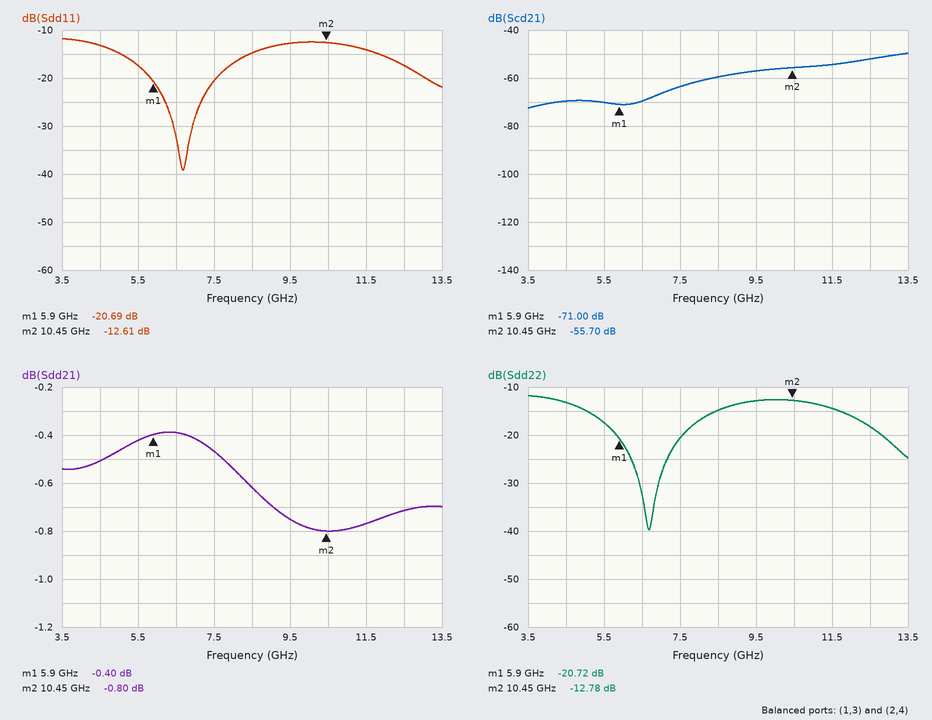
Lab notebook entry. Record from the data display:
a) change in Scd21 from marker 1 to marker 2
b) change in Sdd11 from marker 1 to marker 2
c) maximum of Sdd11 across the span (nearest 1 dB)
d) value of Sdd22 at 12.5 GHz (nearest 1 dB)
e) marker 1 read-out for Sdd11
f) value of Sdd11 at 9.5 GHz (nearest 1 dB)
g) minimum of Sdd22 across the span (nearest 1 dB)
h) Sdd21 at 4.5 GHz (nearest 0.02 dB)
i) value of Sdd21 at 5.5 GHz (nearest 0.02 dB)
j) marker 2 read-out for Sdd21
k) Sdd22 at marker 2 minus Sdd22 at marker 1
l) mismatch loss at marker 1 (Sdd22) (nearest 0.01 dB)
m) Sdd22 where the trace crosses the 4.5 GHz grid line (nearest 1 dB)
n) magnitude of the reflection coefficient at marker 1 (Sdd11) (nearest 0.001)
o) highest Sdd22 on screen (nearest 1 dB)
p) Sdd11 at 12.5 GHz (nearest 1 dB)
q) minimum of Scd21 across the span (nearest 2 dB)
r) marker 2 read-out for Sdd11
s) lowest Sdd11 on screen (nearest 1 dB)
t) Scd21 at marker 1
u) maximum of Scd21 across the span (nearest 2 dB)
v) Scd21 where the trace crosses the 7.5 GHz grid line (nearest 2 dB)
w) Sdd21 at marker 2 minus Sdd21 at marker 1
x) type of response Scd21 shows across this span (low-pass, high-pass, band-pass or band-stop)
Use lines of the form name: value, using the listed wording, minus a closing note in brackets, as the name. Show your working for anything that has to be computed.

change in Scd21 from marker 1 to marker 2: -55.7 − (-71) = 15.30 dB
change in Sdd11 from marker 1 to marker 2: -12.61 − (-20.69) = 8.08 dB
maximum of Sdd11 across the span: -12 dB
value of Sdd22 at 12.5 GHz: -18 dB
marker 1 read-out for Sdd11: -20.69 dB
value of Sdd11 at 9.5 GHz: -13 dB
minimum of Sdd22 across the span: -40 dB
Sdd21 at 4.5 GHz: -0.50 dB
value of Sdd21 at 5.5 GHz: -0.42 dB
marker 2 read-out for Sdd21: -0.80 dB
Sdd22 at marker 2 minus Sdd22 at marker 1: -12.78 − (-20.72) = 7.94 dB
mismatch loss at marker 1 (Sdd22): −10 log10(1 − 10^(-20.72/10)) ≈ 0.04 dB
Sdd22 where the trace crosses the 4.5 GHz grid line: -13 dB
magnitude of the reflection coefficient at marker 1 (Sdd11): 10^(-20.69/20) ≈ 0.092
highest Sdd22 on screen: -12 dB
Sdd11 at 12.5 GHz: -17 dB
minimum of Scd21 across the span: -72 dB
marker 2 read-out for Sdd11: -12.61 dB
lowest Sdd11 on screen: -39 dB
Scd21 at marker 1: -71.00 dB
maximum of Scd21 across the span: -50 dB
Scd21 where the trace crosses the 7.5 GHz grid line: -64 dB
Sdd21 at marker 2 minus Sdd21 at marker 1: -0.8 − (-0.4) = -0.40 dB
type of response Scd21 shows across this span: high-pass
